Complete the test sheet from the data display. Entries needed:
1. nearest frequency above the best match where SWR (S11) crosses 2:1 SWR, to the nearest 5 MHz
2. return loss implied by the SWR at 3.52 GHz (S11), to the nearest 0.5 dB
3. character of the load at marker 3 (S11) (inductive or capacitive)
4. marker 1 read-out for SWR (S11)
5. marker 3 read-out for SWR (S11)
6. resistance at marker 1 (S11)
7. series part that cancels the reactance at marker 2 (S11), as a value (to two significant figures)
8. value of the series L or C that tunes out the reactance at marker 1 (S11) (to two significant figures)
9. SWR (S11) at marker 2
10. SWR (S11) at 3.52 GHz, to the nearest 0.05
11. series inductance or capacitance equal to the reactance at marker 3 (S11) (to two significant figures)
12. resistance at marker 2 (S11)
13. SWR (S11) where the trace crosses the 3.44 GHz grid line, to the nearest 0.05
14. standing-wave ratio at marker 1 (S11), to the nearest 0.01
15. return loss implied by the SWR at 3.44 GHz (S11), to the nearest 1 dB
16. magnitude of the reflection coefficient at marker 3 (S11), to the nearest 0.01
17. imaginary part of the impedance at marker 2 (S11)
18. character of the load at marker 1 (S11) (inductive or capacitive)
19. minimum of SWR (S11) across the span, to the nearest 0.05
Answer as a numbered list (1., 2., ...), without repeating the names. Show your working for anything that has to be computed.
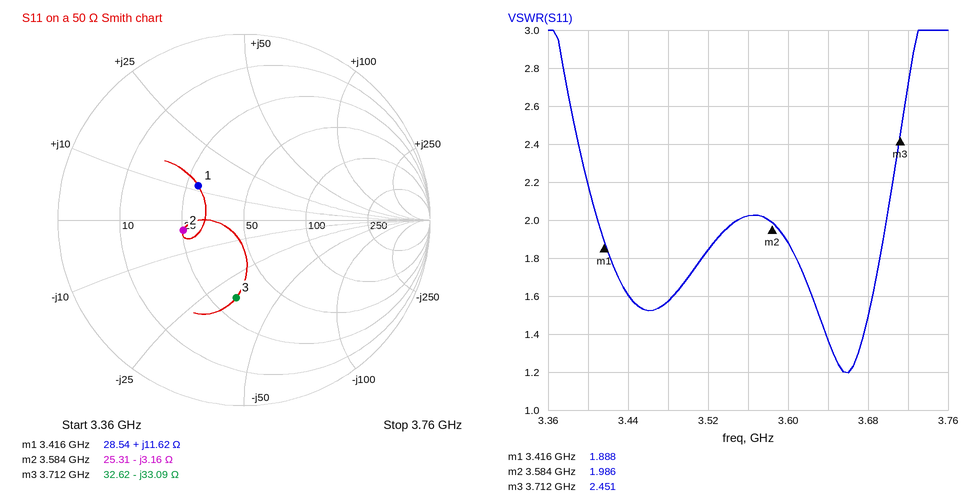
1. 3.700 GHz
2. −20 log10((1.85 − 1)/(1.85 + 1)) ≈ 10.5 dB
3. capacitive
4. 1.888
5. 2.451
6. 28.54 Ω
7. L = 3.16 Ω/(2π × 3.584 GHz) ≈ 140 pH
8. C = 1/(2π × 3.416 GHz × 11.62 Ω) ≈ 4.0 pF
9. 1.986
10. 1.85
11. C = 1/(2π × 3.712 GHz × 33.09 Ω) ≈ 1.3 pF
12. 25.31 Ω
13. 1.60
14. 1.89
15. −20 log10((1.6 − 1)/(1.6 + 1)) ≈ 13 dB
16. 0.42
17. -3.16 Ω
18. inductive
19. 1.20
